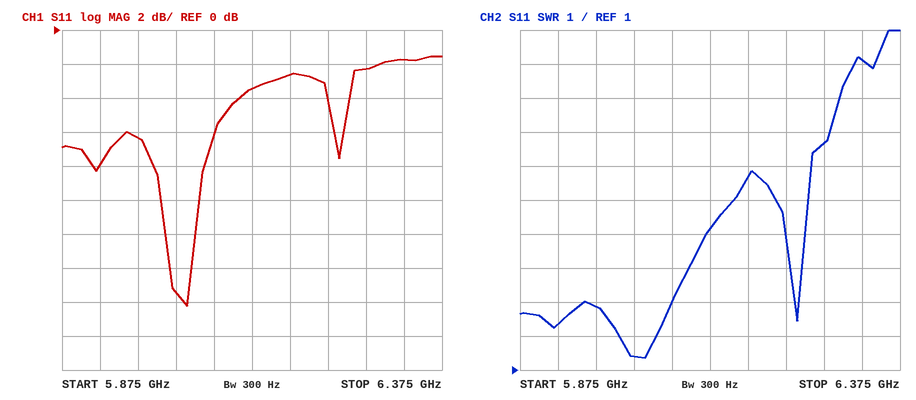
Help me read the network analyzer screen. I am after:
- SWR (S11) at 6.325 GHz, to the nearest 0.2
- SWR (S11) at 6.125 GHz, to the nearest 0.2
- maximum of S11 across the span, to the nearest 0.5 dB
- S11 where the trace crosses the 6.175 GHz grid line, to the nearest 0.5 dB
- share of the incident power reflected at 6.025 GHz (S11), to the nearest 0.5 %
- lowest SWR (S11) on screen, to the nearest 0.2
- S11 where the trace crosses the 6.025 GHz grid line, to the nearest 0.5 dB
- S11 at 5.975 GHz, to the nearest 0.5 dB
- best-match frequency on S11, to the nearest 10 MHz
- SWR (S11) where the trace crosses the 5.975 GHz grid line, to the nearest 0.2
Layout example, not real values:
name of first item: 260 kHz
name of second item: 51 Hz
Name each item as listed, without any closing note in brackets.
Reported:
SWR (S11) at 6.325 GHz, to the nearest 0.2: 10.2
SWR (S11) at 6.125 GHz, to the nearest 0.2: 5.2
maximum of S11 across the span, to the nearest 0.5 dB: -1.5 dB
S11 where the trace crosses the 6.175 GHz grid line, to the nearest 0.5 dB: -2.5 dB
share of the incident power reflected at 6.025 GHz (S11), to the nearest 0.5 %: 3.0 %
lowest SWR (S11) on screen, to the nearest 0.2: 1.4
S11 where the trace crosses the 6.025 GHz grid line, to the nearest 0.5 dB: -15.5 dB
S11 at 5.975 GHz, to the nearest 0.5 dB: -6.5 dB
best-match frequency on S11, to the nearest 10 MHz: 6.04 GHz
SWR (S11) where the trace crosses the 5.975 GHz grid line, to the nearest 0.2: 2.8
